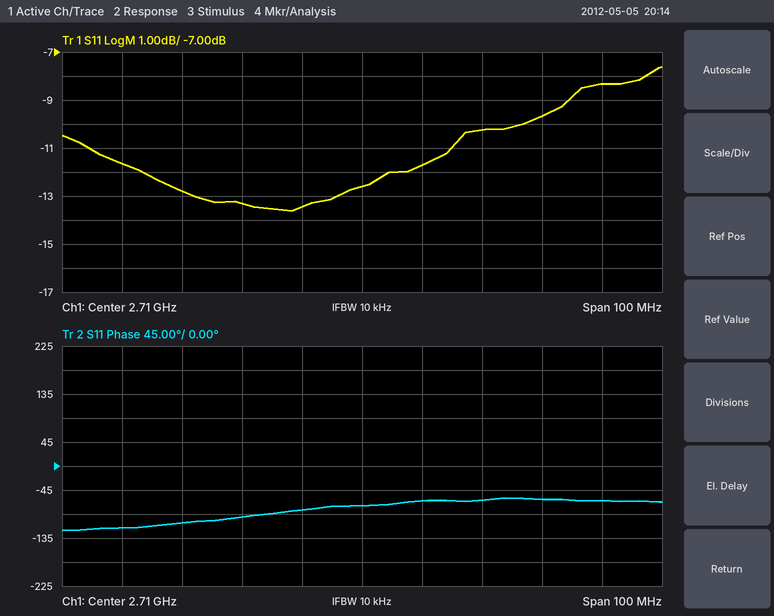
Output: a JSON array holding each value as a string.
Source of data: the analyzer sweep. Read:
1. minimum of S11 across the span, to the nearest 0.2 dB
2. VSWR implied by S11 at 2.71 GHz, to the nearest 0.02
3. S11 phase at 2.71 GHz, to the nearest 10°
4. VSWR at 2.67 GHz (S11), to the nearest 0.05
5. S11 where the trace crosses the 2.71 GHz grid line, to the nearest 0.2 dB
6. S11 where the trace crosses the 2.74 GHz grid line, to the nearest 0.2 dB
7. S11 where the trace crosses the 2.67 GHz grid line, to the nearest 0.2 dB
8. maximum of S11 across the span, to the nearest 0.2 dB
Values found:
["-13.6 dB", "1.62", "-70°", "1.70", "-12.6 dB", "-9.6 dB", "-11.6 dB", "-7.6 dB"]
